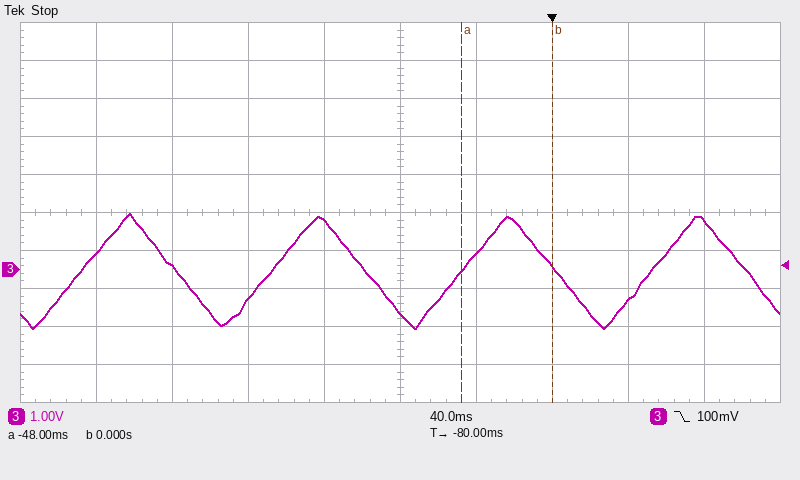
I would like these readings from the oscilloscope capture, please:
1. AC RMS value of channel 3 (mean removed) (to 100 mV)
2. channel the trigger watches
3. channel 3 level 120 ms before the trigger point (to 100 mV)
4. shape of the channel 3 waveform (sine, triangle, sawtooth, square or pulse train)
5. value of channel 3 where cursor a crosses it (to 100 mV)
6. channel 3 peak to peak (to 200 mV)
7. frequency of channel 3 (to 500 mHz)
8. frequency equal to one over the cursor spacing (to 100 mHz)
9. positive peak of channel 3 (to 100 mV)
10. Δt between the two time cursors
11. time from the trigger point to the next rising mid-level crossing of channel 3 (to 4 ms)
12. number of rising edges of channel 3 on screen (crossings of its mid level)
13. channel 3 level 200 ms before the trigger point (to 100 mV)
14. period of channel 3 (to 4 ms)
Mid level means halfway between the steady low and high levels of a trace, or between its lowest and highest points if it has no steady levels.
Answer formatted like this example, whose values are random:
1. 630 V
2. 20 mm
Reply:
1. 900 mV
2. channel 3
3. 1.3 V
4. triangle
5. 0.0 V
6. 3.0 V
7. 10.0 Hz
8. 20.8 Hz
9. 1.5 V
10. 48 ms
11. 52 ms
12. 4
13. 100 mV
14. 100 ms
